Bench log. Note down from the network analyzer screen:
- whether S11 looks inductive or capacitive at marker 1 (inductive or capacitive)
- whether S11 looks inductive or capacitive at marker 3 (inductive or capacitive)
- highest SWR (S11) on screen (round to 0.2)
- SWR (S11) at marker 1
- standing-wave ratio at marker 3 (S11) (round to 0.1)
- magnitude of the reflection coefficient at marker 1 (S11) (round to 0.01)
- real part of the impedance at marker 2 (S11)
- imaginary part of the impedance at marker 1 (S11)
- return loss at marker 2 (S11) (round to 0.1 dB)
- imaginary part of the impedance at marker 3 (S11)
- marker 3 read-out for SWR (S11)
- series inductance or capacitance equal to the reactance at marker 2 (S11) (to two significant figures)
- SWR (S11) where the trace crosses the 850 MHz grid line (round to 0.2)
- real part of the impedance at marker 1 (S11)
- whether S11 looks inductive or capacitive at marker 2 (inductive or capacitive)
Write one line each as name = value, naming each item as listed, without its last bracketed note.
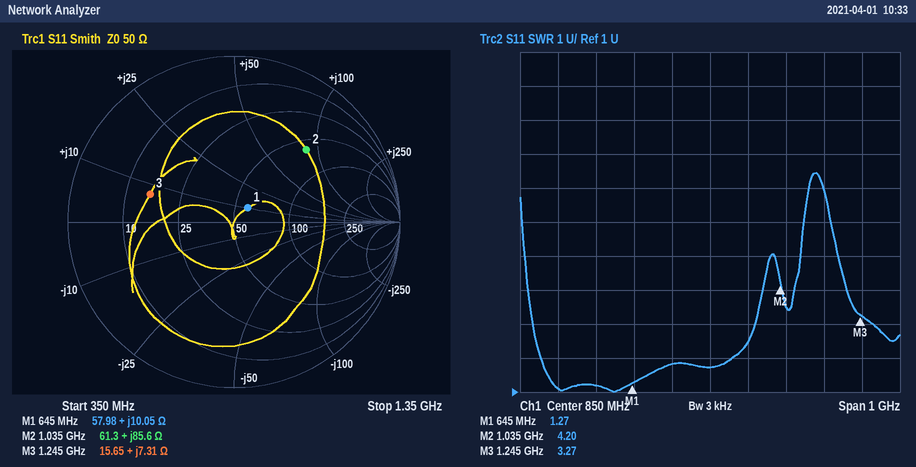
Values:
whether S11 looks inductive or capacitive at marker 1 = inductive
whether S11 looks inductive or capacitive at marker 3 = inductive
highest SWR (S11) on screen = 7.4
SWR (S11) at marker 1 = 1.27
standing-wave ratio at marker 3 (S11) = 3.3
magnitude of the reflection coefficient at marker 1 (S11) = 0.12
real part of the impedance at marker 2 = 61.3 Ω
imaginary part of the impedance at marker 1 = +10.05 Ω
return loss at marker 2 (S11) = 4.2 dB
imaginary part of the impedance at marker 3 = +7.31 Ω
marker 3 read-out for SWR = 3.27
series inductance or capacitance equal to the reactance at marker 2 (S11) = 13 nH
SWR (S11) where the trace crosses the 850 MHz grid line = 1.8
real part of the impedance at marker 1 = 57.98 Ω
whether S11 looks inductive or capacitive at marker 2 = inductive
